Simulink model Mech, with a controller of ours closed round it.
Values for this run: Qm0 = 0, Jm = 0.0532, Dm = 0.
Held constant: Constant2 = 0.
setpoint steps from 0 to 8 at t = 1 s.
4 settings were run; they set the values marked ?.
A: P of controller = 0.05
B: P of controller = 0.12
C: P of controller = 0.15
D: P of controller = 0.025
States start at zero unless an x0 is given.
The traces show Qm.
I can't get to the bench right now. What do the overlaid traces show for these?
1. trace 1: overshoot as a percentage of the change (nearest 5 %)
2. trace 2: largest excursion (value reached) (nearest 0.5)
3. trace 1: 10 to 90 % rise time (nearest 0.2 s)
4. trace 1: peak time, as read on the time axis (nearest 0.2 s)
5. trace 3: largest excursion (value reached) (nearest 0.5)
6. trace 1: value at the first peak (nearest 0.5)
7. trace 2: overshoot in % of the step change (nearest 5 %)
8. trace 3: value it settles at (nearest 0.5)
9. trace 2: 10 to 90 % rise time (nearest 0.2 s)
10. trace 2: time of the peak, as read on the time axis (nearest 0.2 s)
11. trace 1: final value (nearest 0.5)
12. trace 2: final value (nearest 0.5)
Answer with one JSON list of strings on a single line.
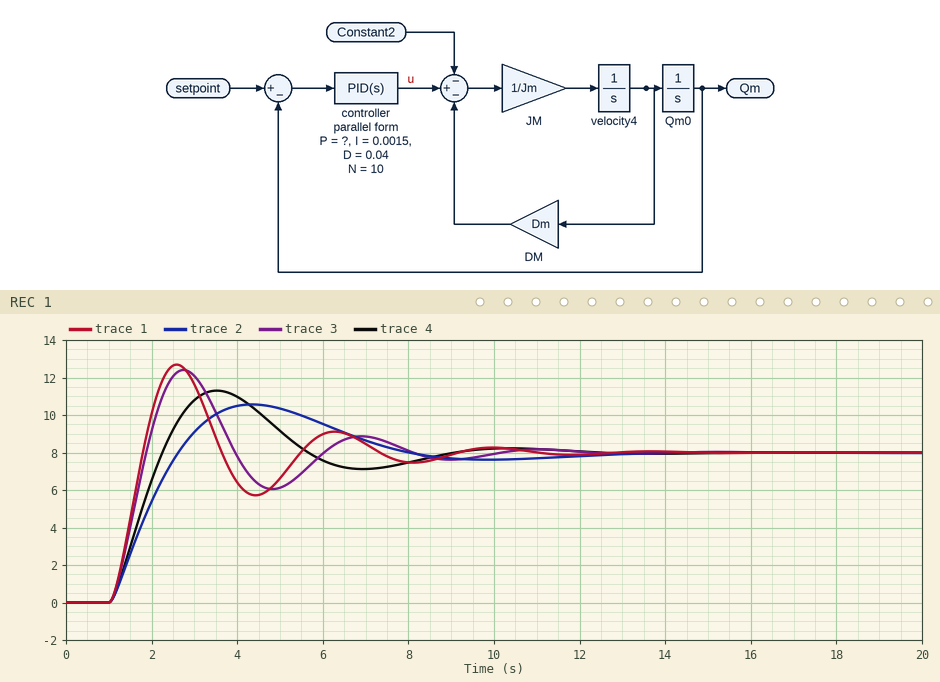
["60 %", "10.5", "0.6 s", "2.6 s", "12.5", "12.5", "30 %", "8.0", "1.2 s", "4.4 s", "8.0", "8.0"]
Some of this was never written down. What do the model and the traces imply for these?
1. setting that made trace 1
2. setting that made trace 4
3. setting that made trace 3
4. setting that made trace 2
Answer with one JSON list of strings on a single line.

["C", "A", "B", "D"]
